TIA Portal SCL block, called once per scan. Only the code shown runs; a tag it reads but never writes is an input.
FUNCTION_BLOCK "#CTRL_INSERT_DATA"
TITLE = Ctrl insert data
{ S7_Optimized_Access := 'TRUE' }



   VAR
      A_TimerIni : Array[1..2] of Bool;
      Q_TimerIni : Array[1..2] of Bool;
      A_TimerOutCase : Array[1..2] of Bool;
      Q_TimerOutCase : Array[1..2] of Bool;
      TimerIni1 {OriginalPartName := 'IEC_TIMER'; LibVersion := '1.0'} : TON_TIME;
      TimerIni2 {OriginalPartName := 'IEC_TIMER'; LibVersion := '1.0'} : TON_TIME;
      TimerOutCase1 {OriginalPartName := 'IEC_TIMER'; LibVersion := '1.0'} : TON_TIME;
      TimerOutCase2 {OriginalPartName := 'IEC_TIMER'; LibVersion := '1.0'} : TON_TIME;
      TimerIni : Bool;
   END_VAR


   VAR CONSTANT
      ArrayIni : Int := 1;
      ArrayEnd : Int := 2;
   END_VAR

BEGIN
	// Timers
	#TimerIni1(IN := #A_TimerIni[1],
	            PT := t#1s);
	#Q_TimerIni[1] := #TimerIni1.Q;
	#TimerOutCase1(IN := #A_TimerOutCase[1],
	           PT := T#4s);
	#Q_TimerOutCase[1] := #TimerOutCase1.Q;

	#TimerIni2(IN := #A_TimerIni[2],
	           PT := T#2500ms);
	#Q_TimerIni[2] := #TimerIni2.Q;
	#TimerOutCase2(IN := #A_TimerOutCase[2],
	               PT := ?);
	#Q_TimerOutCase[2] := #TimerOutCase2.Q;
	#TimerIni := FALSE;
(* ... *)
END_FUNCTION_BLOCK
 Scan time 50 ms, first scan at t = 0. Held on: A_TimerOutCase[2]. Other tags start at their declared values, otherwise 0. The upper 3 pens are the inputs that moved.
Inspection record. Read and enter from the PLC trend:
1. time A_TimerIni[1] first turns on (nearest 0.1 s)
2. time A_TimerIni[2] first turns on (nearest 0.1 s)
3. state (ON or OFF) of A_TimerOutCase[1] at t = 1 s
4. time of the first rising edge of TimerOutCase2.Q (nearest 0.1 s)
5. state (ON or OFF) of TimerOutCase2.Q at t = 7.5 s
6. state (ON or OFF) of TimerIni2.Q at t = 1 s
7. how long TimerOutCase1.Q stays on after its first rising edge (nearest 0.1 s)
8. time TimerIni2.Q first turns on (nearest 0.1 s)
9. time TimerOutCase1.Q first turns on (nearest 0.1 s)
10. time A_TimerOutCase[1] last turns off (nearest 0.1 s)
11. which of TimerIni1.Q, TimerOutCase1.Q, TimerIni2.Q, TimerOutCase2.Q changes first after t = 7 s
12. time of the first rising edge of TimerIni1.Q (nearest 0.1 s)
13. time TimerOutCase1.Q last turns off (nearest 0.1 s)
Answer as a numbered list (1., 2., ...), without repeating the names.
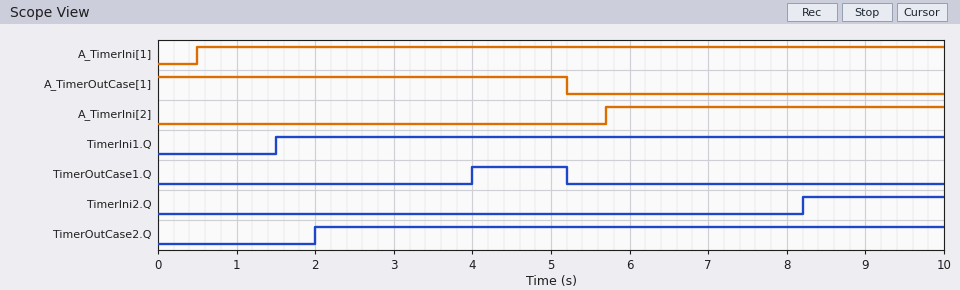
1. 0.5 s
2. 5.7 s
3. ON
4. 2.0 s
5. ON
6. OFF
7. 1.2 s
8. 8.2 s
9. 4.0 s
10. 5.2 s
11. TimerIni2.Q
12. 1.5 s
13. 5.2 s
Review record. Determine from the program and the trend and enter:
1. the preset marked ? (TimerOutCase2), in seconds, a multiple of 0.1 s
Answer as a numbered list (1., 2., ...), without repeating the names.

1. 2.0 s
